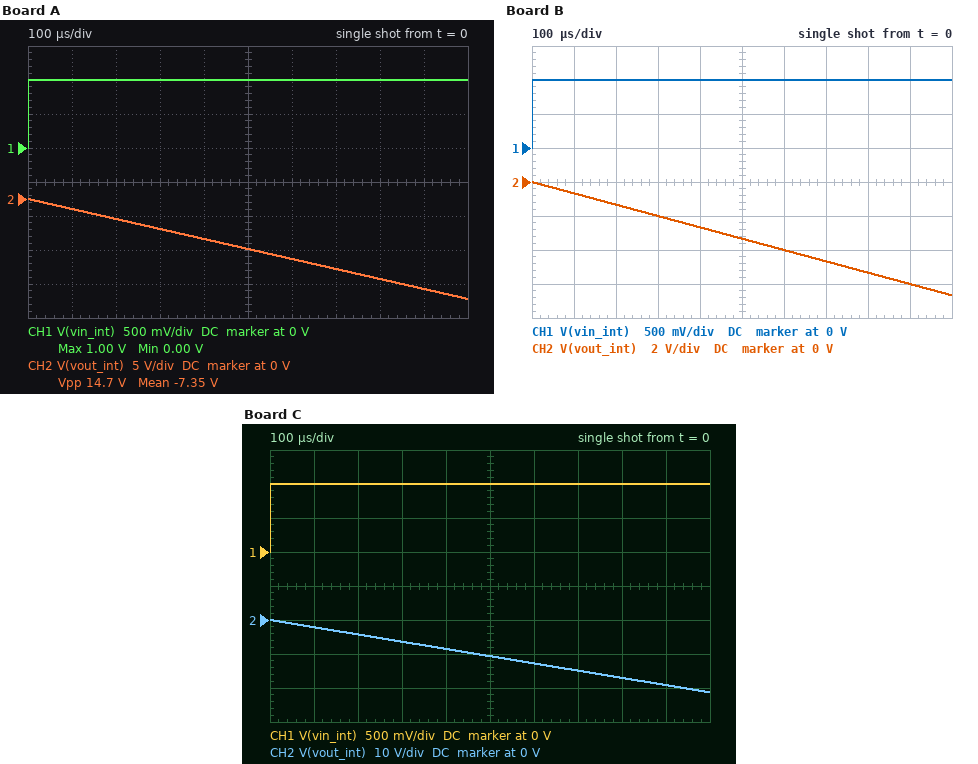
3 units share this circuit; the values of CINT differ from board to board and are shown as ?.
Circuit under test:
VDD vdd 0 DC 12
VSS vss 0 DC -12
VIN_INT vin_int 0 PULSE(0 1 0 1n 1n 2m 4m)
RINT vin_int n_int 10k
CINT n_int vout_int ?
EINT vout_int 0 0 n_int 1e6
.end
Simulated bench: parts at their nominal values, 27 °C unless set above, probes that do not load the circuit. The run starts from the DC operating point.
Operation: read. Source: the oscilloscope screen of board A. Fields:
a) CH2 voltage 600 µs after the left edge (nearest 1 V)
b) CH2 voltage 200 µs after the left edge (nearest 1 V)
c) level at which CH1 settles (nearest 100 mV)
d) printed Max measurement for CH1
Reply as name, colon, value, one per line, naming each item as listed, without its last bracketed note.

CH2 voltage 600 µs after the left edge: -9 V
CH2 voltage 200 µs after the left edge: -3 V
level at which CH1 settles: 1.0 V
printed Max measurement for CH1: 1.00 V
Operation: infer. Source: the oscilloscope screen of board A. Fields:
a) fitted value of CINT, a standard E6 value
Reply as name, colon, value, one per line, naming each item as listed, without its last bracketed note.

fitted value of CINT, a standard E6 value: 6.8 nF
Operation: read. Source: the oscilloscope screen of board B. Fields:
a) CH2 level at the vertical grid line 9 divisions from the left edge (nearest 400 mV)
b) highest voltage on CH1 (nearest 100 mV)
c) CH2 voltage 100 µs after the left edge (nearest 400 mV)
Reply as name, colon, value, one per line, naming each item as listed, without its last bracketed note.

CH2 level at the vertical grid line 9 divisions from the left edge: -6.0 V
highest voltage on CH1: 1.0 V
CH2 voltage 100 µs after the left edge: -800 mV
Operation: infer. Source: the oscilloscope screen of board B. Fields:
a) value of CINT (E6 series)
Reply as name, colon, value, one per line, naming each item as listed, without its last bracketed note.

value of CINT: 15 nF
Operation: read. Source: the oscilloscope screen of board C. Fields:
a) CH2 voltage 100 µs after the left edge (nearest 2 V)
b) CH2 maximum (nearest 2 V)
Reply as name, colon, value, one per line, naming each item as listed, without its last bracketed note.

CH2 voltage 100 µs after the left edge: -2 V
CH2 maximum: 0 V
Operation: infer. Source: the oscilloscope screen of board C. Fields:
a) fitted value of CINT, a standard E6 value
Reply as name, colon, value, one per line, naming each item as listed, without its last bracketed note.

fitted value of CINT, a standard E6 value: 4.7 nF
